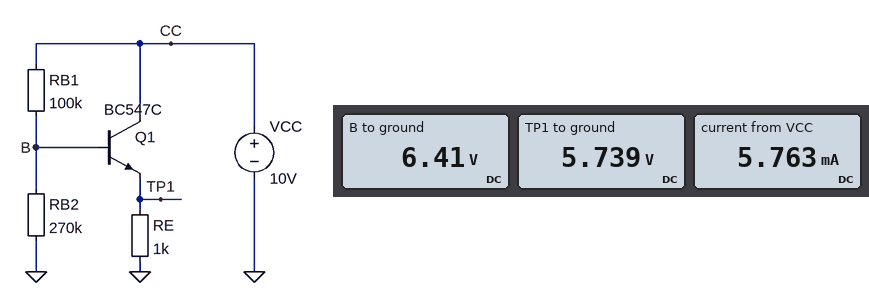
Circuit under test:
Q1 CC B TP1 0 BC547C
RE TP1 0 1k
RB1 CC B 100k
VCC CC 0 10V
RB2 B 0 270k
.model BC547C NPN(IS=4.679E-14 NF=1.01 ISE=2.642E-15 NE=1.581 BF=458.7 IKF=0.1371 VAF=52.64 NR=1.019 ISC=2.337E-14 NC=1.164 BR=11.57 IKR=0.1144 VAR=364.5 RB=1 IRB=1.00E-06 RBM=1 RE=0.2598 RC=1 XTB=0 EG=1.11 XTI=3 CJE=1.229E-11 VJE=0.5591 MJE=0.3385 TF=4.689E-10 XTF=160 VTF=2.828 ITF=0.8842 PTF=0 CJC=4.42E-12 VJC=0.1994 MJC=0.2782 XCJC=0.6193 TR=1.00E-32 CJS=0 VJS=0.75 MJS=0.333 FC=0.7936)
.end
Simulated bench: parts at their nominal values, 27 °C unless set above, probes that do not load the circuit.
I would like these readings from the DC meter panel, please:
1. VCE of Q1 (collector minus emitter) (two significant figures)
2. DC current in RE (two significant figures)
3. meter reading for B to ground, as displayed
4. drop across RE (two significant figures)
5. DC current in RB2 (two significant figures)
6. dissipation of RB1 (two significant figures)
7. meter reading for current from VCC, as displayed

4.3 V
5.7 mA
6.41 V
5.7 V
24 µA
130 µW
5.763 mA
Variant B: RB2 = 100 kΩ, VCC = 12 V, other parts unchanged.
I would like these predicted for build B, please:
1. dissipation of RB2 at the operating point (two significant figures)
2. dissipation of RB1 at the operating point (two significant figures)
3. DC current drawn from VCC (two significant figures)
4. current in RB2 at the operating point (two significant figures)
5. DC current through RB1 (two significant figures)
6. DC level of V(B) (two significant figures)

300 µW
420 µW
4.9 mA
55 µA
65 µA
5.5 V
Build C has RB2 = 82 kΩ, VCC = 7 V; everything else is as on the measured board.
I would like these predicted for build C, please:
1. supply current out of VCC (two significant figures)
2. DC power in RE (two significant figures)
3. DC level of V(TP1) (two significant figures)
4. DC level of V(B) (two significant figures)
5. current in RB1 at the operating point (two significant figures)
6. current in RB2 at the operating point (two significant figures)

2.3 mA
5.3 mW
2.3 V
2.9 V
41 µA
36 µA
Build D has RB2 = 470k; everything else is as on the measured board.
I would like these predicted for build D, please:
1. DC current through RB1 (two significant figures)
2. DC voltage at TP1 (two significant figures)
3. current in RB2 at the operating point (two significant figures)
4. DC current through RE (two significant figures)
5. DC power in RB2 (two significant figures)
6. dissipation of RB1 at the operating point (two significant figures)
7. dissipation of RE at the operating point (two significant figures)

29 µA
6.4 V
15 µA
6.4 mA
110 µW
84 µW
41 mW
